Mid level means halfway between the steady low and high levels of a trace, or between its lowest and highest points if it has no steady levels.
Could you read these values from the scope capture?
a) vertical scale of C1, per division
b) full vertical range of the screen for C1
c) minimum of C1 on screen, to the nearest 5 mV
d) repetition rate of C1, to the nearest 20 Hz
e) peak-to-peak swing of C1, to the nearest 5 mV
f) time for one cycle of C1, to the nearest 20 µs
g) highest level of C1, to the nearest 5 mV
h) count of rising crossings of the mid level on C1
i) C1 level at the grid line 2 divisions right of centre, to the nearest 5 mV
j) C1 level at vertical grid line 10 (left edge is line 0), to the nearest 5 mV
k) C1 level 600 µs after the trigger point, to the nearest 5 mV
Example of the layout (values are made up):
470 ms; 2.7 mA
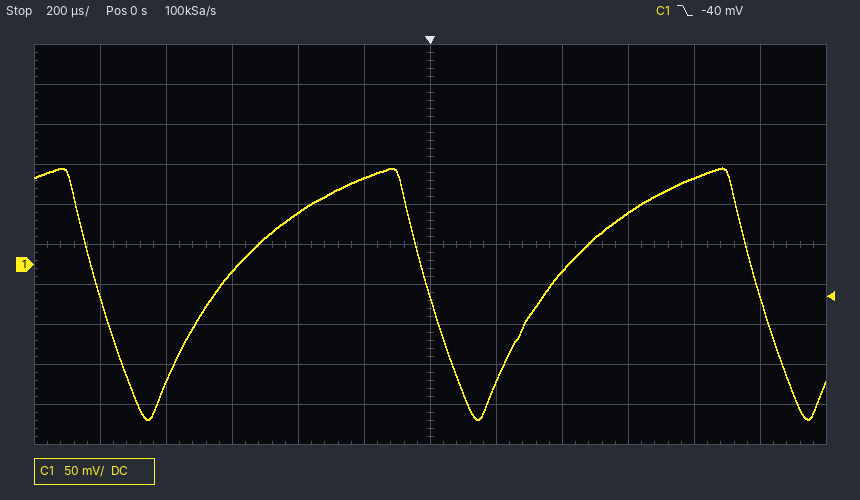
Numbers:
50 mV; 500 mV; -195 mV; 1.00 kHz; 315 mV; 1.00 ms; 120 mV; 2; -10 mV; 110 mV; 65 mV
